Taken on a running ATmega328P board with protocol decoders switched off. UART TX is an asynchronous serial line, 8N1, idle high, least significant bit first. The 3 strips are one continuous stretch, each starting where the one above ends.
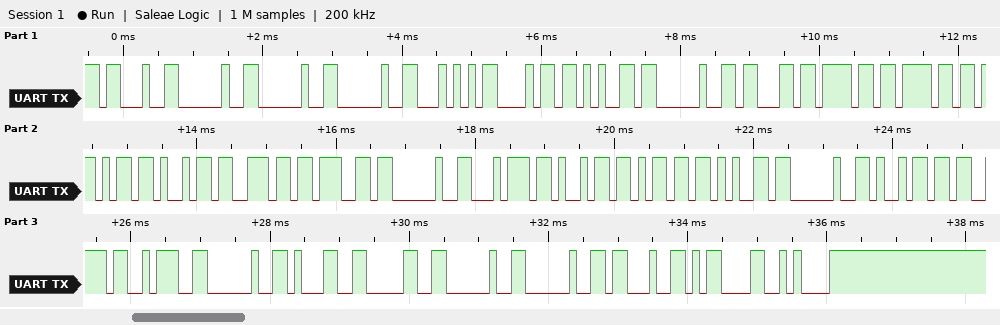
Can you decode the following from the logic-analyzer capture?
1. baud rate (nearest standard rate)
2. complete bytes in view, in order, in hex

9600 baud
23 20 20 20 54 68 65 20 63 6F 6F 6B 69 6E 67 20 74 69 6D 65 20 69 73 3A 20 31 30 20 20 23 0D 0A
